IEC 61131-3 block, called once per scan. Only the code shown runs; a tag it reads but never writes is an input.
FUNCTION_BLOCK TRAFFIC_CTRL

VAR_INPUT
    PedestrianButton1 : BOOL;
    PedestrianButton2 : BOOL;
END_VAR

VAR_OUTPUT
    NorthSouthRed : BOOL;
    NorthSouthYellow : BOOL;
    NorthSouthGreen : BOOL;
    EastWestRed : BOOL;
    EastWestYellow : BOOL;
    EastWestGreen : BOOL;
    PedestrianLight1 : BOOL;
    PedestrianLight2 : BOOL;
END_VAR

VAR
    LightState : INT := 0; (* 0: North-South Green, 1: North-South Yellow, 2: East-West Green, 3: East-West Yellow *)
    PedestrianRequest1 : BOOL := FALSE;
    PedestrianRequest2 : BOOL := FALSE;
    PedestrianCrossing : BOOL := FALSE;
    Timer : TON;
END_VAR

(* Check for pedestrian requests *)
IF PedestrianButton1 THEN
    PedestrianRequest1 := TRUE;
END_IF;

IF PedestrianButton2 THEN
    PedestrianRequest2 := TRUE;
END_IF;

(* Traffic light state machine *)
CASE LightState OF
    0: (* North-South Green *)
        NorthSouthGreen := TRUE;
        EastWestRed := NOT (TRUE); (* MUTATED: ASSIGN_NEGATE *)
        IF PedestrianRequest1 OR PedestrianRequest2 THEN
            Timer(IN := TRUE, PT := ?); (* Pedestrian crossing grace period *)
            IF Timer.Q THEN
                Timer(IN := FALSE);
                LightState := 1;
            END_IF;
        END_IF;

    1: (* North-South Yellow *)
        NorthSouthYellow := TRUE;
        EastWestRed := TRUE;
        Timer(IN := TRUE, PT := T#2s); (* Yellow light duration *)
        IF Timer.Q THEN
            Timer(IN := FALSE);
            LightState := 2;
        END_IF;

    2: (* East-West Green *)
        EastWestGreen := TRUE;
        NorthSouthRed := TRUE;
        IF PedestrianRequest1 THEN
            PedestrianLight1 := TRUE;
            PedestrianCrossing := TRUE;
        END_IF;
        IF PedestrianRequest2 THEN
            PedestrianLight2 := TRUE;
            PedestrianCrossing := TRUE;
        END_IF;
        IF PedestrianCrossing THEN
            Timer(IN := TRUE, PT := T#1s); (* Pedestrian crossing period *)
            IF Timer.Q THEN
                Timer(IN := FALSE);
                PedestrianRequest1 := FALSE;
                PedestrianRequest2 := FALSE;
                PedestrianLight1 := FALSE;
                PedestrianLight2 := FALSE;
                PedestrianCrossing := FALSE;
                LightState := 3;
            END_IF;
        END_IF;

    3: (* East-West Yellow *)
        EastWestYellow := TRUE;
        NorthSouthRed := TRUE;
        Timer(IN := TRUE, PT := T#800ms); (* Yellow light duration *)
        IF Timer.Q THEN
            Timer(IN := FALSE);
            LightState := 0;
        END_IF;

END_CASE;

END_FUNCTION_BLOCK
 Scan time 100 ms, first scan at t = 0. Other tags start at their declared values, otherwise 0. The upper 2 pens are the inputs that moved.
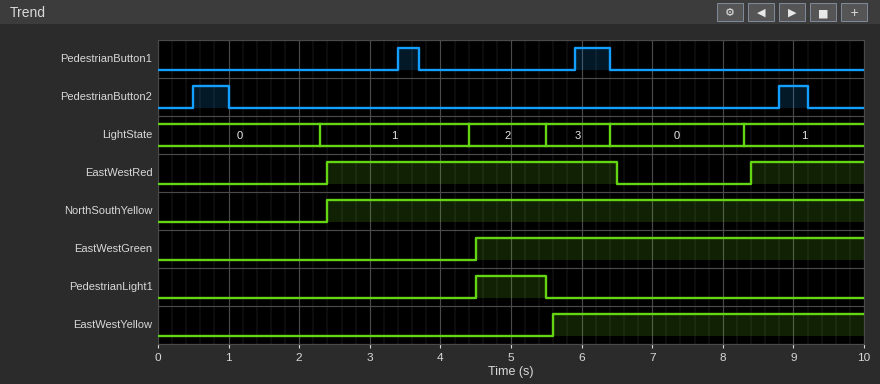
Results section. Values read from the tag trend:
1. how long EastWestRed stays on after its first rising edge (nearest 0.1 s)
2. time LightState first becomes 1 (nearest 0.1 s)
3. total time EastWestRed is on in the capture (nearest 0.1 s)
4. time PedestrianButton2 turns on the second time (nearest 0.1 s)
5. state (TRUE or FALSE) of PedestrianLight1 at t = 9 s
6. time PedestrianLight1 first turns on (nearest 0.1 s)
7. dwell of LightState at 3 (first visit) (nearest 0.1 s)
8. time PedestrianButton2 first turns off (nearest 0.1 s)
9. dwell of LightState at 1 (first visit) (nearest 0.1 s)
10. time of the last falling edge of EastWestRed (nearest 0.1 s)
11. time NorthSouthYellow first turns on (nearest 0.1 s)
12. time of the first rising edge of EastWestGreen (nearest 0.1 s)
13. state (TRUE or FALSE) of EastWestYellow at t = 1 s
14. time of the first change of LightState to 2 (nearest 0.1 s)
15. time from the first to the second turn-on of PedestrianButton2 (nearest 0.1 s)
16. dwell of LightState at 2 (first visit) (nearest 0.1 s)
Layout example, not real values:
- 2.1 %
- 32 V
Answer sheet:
- 4.1 s
- 2.3 s
- 5.7 s
- 8.8 s
- FALSE
- 4.5 s
- 0.9 s
- 1.0 s
- 2.1 s
- 6.5 s
- 2.4 s
- 4.5 s
- FALSE
- 4.4 s
- 8.3 s
- 1.1 s
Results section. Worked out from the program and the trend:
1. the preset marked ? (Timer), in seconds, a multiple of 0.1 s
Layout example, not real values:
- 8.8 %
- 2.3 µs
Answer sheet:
- 1.8 s
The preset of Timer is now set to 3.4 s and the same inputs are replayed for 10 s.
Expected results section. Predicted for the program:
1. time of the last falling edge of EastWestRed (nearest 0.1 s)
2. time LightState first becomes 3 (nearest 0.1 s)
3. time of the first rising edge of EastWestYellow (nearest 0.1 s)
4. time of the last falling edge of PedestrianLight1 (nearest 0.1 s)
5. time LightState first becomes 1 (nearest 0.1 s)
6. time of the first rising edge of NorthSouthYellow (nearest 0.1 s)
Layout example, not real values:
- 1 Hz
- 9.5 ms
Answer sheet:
- 8.1 s
- 7.1 s
- 7.2 s
- 7.1 s
- 3.9 s
- 4.0 s
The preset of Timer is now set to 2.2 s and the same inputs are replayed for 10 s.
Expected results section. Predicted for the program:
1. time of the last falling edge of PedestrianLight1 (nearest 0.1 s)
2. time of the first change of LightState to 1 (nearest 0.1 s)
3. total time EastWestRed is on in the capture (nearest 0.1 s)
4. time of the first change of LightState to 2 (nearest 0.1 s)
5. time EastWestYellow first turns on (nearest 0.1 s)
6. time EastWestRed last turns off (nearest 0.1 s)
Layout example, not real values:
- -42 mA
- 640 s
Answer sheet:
- 5.9 s
- 2.7 s
- 4.9 s
- 4.8 s
- 6.0 s
- 6.9 s
